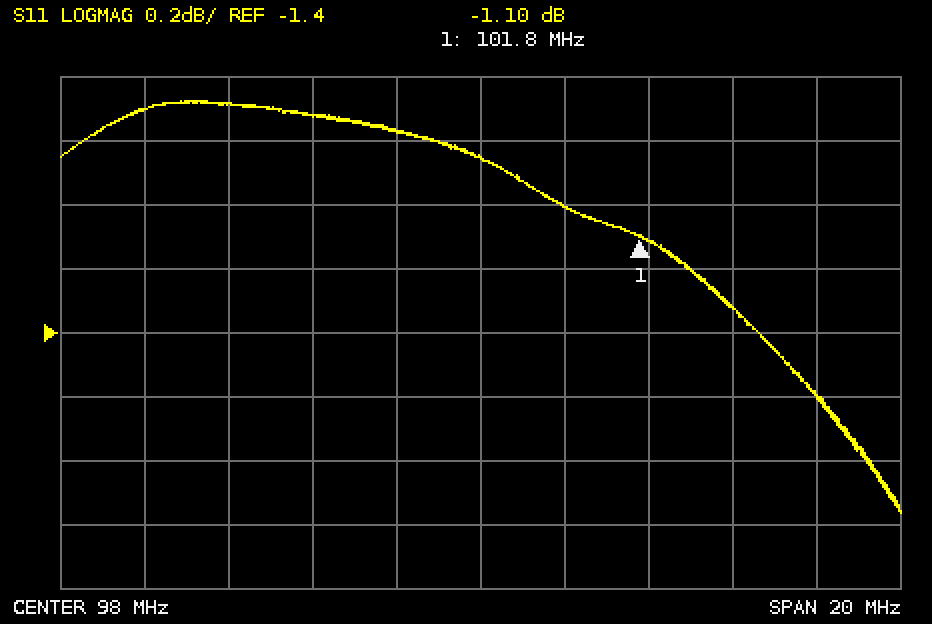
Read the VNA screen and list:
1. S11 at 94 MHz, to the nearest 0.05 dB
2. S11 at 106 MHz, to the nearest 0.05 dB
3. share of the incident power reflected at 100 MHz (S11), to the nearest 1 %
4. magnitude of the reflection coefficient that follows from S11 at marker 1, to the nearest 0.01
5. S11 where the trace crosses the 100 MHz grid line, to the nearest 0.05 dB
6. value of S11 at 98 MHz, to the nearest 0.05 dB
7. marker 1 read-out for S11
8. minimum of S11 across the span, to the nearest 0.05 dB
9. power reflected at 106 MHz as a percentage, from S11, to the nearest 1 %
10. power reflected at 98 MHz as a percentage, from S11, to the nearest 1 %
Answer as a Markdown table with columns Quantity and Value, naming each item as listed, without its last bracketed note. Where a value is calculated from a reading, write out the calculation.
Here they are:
| Quantity | Value |
|---|---|
| S11 at 94 MHz, to the nearest 0.05 dB | -0.70 dB |
| S11 at 106 MHz, to the nearest 0.05 dB | -1.60 dB |
| share of the incident power reflected at 100 MHz (S11), to the nearest 1 % | 10^(-1/10) ≈ 79 % |
| magnitude of the reflection coefficient that follows from S11 at marker 1, to the nearest 0.01 | 10^(-1.1/20) ≈ 0.88 |
| S11 where the trace crosses the 100 MHz grid line, to the nearest 0.05 dB | -1.00 dB |
| value of S11 at 98 MHz, to the nearest 0.05 dB | -0.85 dB |
| marker 1 read-out for S11 | -1.10 dB |
| minimum of S11 across the span, to the nearest 0.05 dB | -1.95 dB |
| power reflected at 106 MHz as a percentage, from S11, to the nearest 1 % | 10^(-1.6/10) ≈ 69 % |
| power reflected at 98 MHz as a percentage, from S11, to the nearest 1 % | 10^(-0.85/10) ≈ 82 % |
